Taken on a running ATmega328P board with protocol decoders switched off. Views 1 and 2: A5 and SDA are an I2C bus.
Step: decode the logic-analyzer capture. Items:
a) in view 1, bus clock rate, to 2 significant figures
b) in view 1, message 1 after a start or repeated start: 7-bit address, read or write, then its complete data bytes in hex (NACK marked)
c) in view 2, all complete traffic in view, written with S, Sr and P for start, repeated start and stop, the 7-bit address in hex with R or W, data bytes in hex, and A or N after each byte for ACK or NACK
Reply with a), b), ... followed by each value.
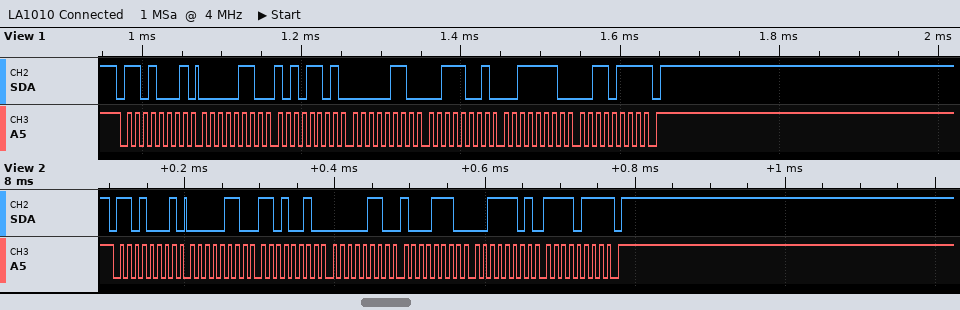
a) 100 kHz
b) 0x68 read: 06 AD 06 39 3E 37 NACK
c) S 68R A 06 A D2 A 06 A 8E A 3D A F7 N P
